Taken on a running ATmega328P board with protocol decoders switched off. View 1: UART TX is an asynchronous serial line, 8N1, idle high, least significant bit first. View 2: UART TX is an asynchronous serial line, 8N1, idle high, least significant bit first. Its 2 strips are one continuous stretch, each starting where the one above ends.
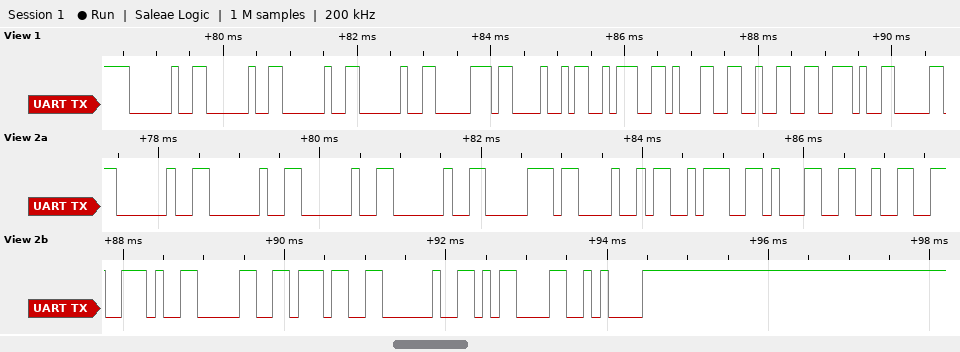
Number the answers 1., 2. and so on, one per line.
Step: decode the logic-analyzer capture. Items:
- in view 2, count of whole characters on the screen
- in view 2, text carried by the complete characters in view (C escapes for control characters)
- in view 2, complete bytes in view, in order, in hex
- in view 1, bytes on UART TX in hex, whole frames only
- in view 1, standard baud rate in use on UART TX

1. 15
2. "    pH:12.07 \r\n"
3. 0x20 0x20 0x20 0x20 0x70 0x48 0x3A 0x31 0x32 0x2E 0x30 0x37 0x20 0x0D 0x0A
4. 0x20 0x20 0x20 0x20 0x70 0x48 0x3A 0x31 0x32 0x2E
5. 9600 baud
